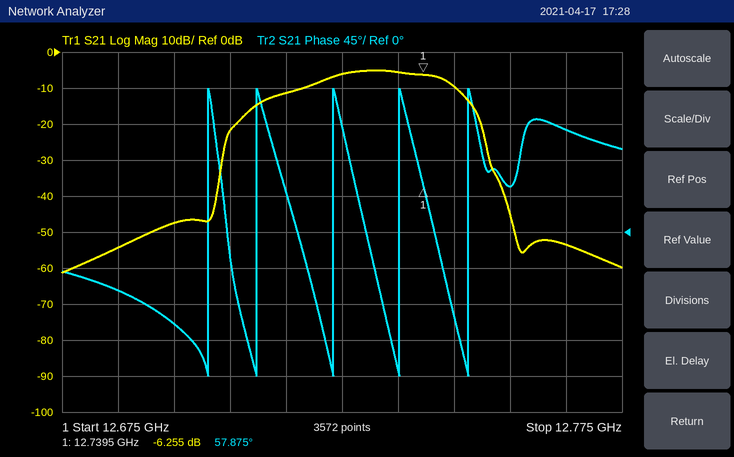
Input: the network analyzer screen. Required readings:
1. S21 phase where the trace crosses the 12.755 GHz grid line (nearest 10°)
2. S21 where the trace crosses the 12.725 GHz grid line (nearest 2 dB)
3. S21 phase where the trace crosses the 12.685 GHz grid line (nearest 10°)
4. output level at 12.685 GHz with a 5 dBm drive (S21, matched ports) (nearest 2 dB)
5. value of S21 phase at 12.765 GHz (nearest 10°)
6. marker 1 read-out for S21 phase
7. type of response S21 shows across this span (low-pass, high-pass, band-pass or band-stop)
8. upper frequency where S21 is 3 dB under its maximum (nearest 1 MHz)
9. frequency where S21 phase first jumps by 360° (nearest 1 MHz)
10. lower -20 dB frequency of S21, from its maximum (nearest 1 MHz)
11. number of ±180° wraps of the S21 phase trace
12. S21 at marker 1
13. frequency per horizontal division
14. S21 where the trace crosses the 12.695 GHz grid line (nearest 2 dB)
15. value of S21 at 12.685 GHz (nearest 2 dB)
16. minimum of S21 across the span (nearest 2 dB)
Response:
60°
-6 dB
-70°
-50 dBm
130°
57.875°
band-pass
12.744 GHz
12.701 GHz
12.704 GHz
5
-6.255 dB
10 MHz
-48 dB
-54 dB
-62 dB
